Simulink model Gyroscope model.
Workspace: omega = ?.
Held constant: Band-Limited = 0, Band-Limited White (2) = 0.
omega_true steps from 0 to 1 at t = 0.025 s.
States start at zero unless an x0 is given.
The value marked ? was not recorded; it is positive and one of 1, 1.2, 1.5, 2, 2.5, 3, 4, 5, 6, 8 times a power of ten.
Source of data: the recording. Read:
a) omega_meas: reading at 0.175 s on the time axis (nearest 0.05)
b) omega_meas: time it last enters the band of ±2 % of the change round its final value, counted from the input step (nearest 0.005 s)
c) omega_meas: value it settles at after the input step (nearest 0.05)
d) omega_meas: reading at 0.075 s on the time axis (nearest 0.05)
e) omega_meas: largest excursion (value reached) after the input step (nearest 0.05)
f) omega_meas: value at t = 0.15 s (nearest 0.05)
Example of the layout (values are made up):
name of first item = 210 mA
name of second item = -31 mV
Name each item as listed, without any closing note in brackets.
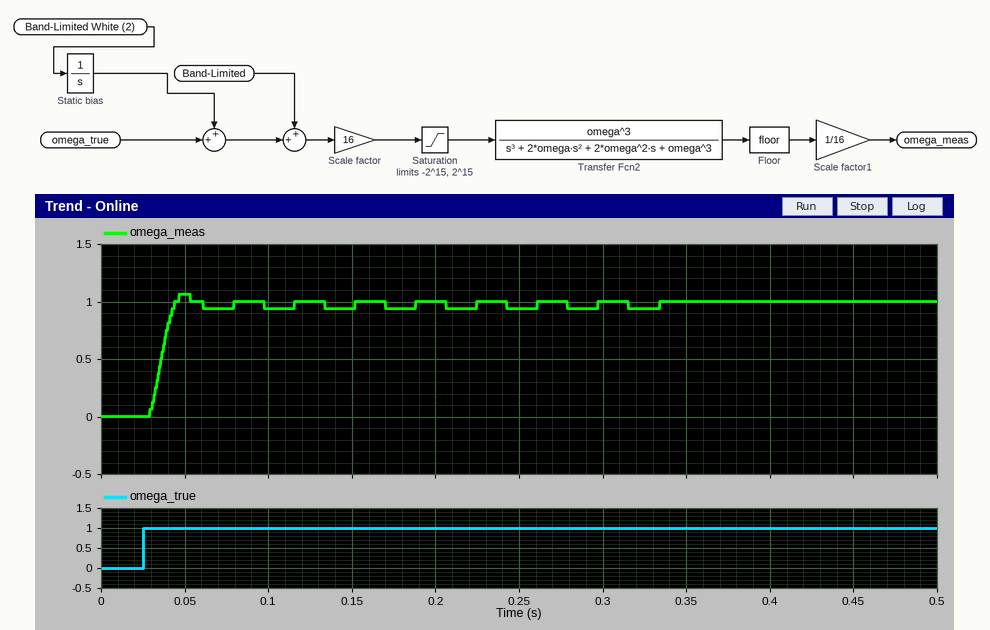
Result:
omega_meas: reading at 0.175 s on the time axis = 0.95
omega_meas: time it last enters the band of ±2 % of the change round its final value, counted from the input step = 0.310 s
omega_meas: value it settles at after the input step = 1.00
omega_meas: reading at 0.075 s on the time axis = 0.95
omega_meas: largest excursion (value reached) after the input step = 1.05
omega_meas: value at t = 0.15 s = 0.95
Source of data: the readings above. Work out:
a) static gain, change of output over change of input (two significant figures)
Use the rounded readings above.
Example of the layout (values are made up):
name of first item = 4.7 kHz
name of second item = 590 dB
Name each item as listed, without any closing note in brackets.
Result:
static gain, change of output over change of input = 1.0
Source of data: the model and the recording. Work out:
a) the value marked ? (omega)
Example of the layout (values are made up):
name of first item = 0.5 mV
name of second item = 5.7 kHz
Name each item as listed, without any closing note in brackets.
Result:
the value marked ? = 200
